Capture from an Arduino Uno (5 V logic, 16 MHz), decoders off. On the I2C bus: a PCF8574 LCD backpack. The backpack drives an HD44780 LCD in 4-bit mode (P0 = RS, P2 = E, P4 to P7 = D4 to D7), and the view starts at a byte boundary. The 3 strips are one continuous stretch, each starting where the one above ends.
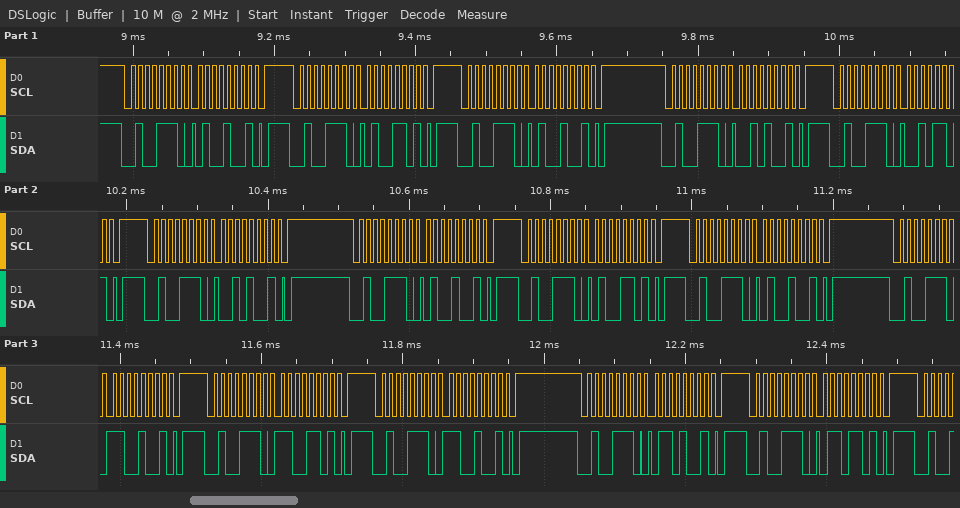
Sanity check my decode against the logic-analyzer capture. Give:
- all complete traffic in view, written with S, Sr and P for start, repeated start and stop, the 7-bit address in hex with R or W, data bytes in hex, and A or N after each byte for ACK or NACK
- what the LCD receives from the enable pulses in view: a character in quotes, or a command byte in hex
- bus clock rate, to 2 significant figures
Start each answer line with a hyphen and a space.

- S 27W A 49 A P S 27W A 4D A P S 27W A 49 A P S 27W A 29 A P S 27W A 2D A P S 27W A 29 A P S 27W A 49 A P S 27W A 4D A P S 27W A 49 A P S 27W A C9 A P S 27W A CD A P S 27W A C9 A P S 27W A 69 A P S 27W A 6D A P
- 'B' 'L'
- 100 kHz
